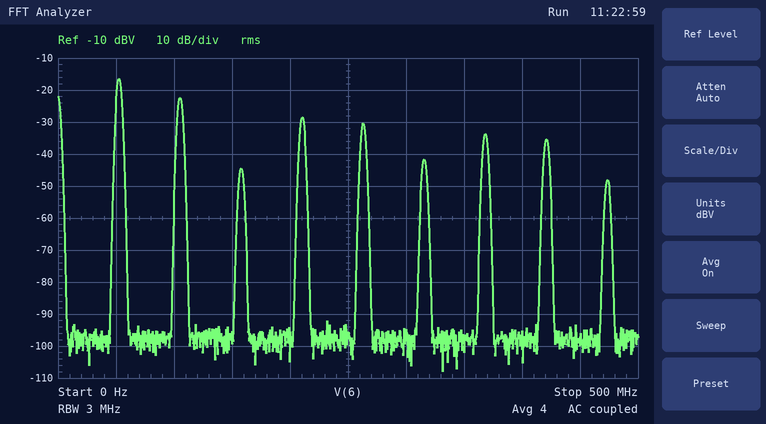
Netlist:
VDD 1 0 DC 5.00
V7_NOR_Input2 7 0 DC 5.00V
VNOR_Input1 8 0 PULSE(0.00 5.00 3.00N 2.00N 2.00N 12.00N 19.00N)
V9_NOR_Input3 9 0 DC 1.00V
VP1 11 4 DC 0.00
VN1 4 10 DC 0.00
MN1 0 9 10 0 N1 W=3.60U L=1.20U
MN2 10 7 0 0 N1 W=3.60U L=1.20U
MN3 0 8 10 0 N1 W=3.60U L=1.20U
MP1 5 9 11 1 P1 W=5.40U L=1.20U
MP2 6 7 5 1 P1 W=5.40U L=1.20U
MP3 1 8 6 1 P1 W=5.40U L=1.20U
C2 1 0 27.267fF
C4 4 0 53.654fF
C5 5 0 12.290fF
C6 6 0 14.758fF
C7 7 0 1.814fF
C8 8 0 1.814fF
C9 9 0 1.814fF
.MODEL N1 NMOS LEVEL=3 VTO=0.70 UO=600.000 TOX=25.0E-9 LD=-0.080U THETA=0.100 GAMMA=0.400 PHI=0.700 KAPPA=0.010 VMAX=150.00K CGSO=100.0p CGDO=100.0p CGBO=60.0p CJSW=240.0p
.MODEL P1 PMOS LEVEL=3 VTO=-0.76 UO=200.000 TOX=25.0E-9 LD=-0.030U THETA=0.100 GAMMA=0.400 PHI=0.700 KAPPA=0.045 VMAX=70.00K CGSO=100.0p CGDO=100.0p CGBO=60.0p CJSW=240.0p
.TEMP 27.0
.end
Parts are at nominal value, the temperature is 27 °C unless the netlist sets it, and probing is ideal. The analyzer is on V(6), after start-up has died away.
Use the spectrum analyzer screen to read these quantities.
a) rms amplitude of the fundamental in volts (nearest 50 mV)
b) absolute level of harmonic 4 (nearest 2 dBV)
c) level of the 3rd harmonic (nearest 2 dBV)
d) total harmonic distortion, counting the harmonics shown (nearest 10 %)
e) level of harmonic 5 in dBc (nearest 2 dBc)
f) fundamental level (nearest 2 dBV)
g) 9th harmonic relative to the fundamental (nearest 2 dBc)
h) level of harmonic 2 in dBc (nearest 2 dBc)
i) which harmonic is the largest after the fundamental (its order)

150 mV
-28 dBV
-44 dBV
60 %
-14 dBc
-16 dBV
-32 dBc
-6 dBc
2
